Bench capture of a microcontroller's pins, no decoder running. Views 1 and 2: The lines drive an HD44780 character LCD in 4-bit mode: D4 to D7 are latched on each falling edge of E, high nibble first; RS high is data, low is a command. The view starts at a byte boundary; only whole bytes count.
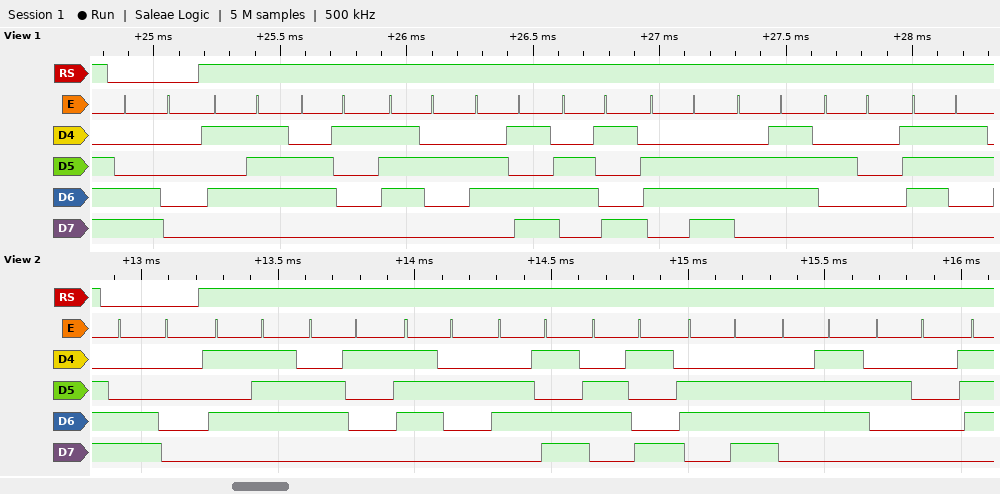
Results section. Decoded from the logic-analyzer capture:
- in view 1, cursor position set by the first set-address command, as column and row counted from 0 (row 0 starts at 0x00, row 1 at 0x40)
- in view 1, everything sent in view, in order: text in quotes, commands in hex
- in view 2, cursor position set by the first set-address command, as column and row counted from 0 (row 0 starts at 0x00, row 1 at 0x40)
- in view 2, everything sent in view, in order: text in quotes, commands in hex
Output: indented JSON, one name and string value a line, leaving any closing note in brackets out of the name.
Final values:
{
  "in view 1, cursor position set by the first set-address command, as column and row counted from 0": "column 0, row 1",
  "in view 1, everything sent in view, in order: text in quotes, commands in hex": "0xC0 \"Warming s\"",
  "in view 2, cursor position set by the first set-address command, as column and row counted from 0": "column 0, row 1",
  "in view 2, everything sent in view, in order: text in quotes, commands in hex": "0xC0 \"Warming \""
}
